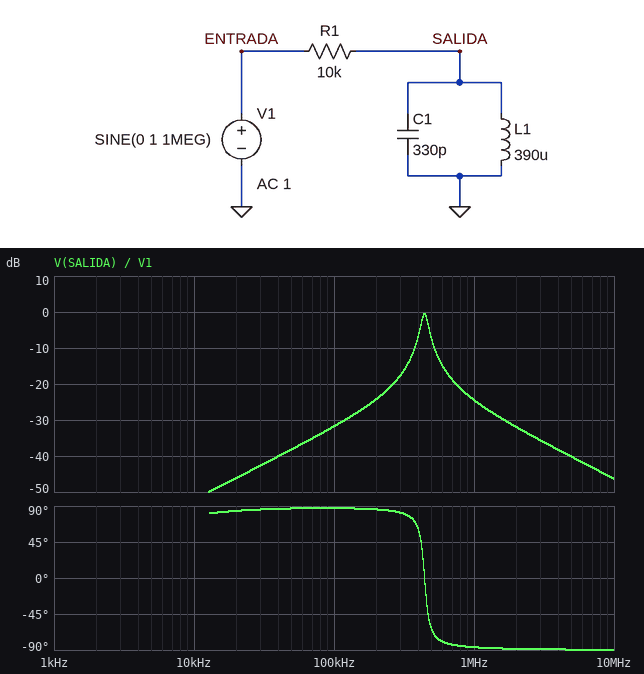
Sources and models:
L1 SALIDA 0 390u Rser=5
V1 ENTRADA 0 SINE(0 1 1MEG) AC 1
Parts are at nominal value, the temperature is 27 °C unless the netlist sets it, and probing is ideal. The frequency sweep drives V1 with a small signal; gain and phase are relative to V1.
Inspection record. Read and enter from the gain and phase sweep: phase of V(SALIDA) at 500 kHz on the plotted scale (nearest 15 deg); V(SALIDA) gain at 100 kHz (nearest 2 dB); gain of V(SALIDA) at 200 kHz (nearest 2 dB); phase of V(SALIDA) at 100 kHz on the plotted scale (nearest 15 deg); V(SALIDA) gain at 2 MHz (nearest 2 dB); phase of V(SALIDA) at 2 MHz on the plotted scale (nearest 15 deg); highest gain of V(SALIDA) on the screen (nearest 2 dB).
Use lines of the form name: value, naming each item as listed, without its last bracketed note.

phase of V(SALIDA) at 500 kHz on the plotted scale: -60 deg
V(SALIDA) gain at 100 kHz: -32 dB
gain of V(SALIDA) at 200 kHz: -24 dB
phase of V(SALIDA) at 100 kHz on the plotted scale: 90 deg
V(SALIDA) gain at 2 MHz: -32 dB
phase of V(SALIDA) at 2 MHz on the plotted scale: -90 deg
highest gain of V(SALIDA) on the screen: 0 dB
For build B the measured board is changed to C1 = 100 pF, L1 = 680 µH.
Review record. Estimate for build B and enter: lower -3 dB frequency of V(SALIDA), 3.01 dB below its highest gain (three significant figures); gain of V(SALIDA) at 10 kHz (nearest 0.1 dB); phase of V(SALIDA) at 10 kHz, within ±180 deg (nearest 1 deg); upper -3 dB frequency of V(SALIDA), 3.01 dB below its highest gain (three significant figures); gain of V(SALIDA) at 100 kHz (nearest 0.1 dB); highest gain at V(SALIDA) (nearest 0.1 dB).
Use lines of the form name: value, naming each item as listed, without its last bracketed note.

lower -3 dB frequency of V(SALIDA), 3.01 dB below its highest gain: 536 kHz
gain of V(SALIDA) at 10 kHz: -47.3 dB
phase of V(SALIDA) at 10 kHz, within ±180 deg: 83 deg
upper -3 dB frequency of V(SALIDA), 3.01 dB below its highest gain: 696 kHz
gain of V(SALIDA) at 100 kHz: -27.2 dB
highest gain at V(SALIDA): -0.1 dB
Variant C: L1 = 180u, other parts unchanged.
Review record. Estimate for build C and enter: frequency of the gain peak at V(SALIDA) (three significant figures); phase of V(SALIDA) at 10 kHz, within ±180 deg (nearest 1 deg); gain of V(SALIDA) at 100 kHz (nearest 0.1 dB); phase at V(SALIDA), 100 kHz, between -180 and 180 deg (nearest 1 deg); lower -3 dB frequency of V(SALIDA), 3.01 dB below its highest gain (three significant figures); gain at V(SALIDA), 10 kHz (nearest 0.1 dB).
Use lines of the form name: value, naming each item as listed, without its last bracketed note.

frequency of the gain peak at V(SALIDA): 653 kHz
phase of V(SALIDA) at 10 kHz, within ±180 deg: 66 deg
gain of V(SALIDA) at 100 kHz: -38.7 dB
phase at V(SALIDA), 100 kHz, between -180 and 180 deg: 87 deg
lower -3 dB frequency of V(SALIDA), 3.01 dB below its highest gain: 627 kHz
gain at V(SALIDA), 10 kHz: -58.2 dB
